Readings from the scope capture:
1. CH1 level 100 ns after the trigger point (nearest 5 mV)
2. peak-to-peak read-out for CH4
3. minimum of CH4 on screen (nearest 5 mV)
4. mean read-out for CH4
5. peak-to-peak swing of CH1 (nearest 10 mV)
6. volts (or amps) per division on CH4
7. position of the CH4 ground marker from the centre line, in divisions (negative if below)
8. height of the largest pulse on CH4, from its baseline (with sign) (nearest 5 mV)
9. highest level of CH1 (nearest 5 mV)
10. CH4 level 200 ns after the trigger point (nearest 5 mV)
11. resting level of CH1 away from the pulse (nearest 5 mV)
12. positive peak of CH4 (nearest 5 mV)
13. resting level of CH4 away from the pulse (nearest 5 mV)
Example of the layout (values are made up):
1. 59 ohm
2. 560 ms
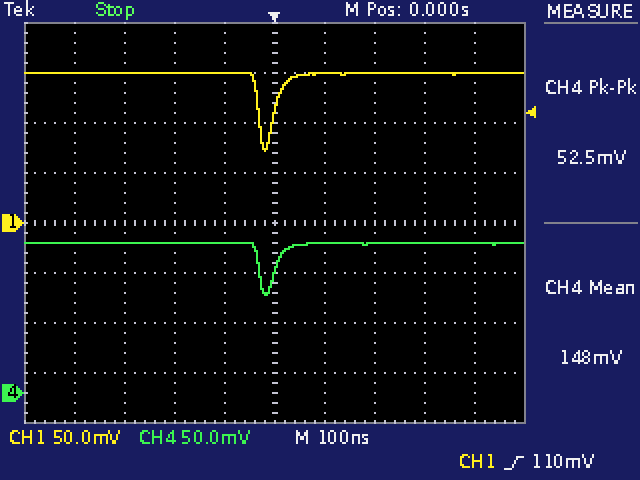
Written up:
1. 150 mV
2. 52.5 mV
3. 100 mV
4. 148 mV
5. 80 mV
6. 50 mV
7. -3.4 div
8. -50 mV
9. 150 mV
10. 150 mV
11. 150 mV
12. 150 mV
13. 150 mV
